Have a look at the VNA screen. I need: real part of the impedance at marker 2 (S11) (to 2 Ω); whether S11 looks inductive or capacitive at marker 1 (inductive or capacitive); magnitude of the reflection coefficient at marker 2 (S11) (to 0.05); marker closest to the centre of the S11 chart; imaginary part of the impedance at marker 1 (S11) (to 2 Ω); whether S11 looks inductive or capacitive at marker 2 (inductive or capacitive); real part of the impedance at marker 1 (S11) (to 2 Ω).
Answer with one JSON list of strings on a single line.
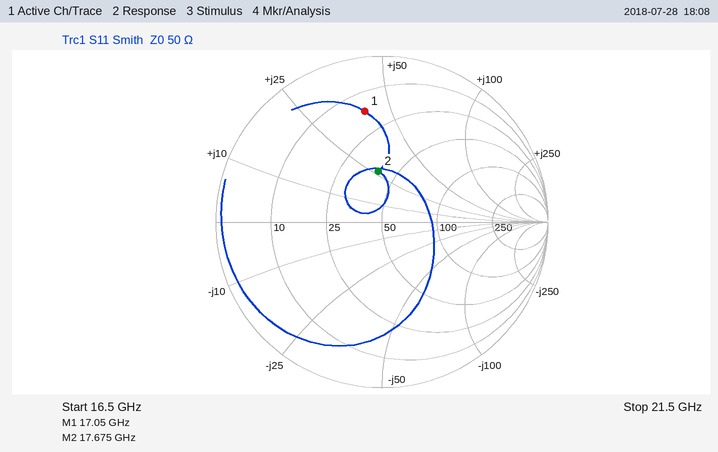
["40 Ω", "inductive", "0.30", "marker 2", "+40 Ω", "inductive", "16 Ω"]
